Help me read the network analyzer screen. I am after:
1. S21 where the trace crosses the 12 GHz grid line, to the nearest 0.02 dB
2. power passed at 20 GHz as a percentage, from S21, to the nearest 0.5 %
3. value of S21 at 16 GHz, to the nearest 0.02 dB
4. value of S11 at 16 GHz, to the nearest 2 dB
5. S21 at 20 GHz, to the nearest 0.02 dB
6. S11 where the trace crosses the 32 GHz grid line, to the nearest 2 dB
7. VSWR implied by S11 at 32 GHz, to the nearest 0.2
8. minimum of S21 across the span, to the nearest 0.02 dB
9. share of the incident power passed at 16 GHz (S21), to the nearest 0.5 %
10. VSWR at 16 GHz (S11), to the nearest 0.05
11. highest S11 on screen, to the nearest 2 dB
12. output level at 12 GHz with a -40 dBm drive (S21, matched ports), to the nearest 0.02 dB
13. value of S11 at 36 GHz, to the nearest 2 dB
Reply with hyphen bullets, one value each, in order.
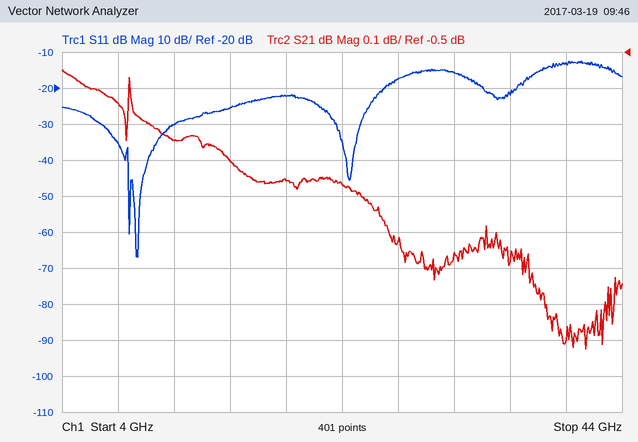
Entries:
- -0.74 dB
- 82.0 %
- -0.80 dB
- -26 dB
- -0.86 dB
- -16 dB
- 1.4
- -1.32 dB
- 83.0 %
- 1.10
- -12 dB
- -40.74 dBm
- -22 dB
